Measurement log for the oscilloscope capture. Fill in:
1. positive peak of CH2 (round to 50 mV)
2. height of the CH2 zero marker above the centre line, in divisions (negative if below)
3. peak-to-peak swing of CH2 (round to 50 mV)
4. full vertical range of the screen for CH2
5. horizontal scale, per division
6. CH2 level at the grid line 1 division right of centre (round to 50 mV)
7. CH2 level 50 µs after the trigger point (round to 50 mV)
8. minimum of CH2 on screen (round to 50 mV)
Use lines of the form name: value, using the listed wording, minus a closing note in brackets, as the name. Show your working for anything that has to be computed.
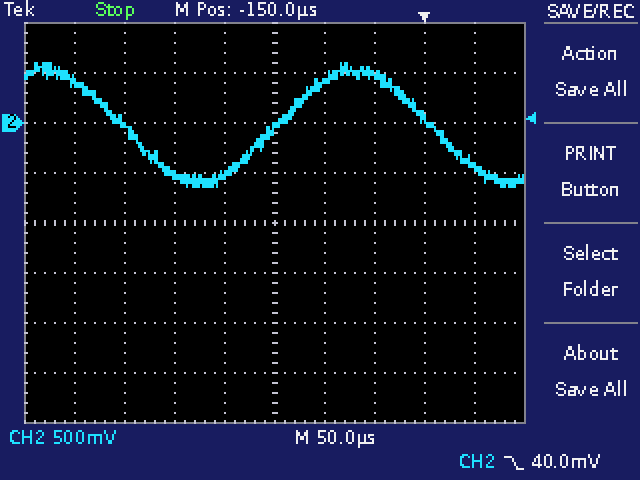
positive peak of CH2: 600 mV
height of the CH2 zero marker above the centre line, in divisions: +2.0 div
peak-to-peak swing of CH2: 600 mV − (-650 mV) = 1.25 V
full vertical range of the screen for CH2: 4 V
horizontal scale, per division: 50 µs
CH2 level at the grid line 1 division right of centre: 400 mV
CH2 level 50 µs after the trigger point: -450 mV
minimum of CH2 on screen: -650 mV
